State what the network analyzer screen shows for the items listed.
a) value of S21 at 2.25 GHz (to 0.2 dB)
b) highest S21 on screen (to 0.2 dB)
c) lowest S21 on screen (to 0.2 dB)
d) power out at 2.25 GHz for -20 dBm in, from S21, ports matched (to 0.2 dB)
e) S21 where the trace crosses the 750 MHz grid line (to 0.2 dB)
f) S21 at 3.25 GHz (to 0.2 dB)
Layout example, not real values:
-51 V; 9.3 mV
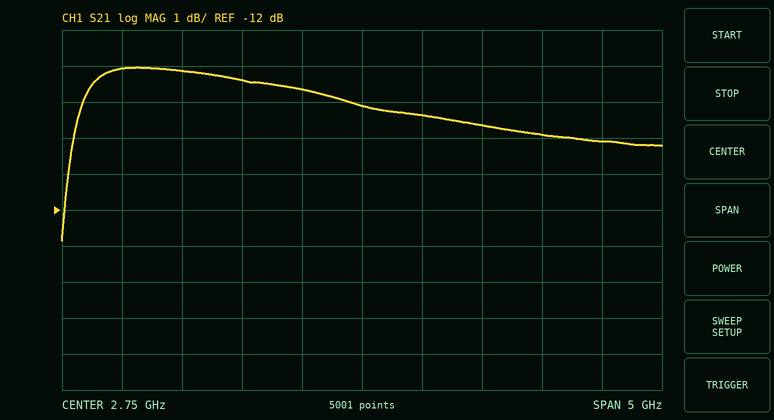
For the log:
-8.6 dB; -8.0 dB; -12.8 dB; -28.6 dBm; -8.0 dB; -9.4 dB
